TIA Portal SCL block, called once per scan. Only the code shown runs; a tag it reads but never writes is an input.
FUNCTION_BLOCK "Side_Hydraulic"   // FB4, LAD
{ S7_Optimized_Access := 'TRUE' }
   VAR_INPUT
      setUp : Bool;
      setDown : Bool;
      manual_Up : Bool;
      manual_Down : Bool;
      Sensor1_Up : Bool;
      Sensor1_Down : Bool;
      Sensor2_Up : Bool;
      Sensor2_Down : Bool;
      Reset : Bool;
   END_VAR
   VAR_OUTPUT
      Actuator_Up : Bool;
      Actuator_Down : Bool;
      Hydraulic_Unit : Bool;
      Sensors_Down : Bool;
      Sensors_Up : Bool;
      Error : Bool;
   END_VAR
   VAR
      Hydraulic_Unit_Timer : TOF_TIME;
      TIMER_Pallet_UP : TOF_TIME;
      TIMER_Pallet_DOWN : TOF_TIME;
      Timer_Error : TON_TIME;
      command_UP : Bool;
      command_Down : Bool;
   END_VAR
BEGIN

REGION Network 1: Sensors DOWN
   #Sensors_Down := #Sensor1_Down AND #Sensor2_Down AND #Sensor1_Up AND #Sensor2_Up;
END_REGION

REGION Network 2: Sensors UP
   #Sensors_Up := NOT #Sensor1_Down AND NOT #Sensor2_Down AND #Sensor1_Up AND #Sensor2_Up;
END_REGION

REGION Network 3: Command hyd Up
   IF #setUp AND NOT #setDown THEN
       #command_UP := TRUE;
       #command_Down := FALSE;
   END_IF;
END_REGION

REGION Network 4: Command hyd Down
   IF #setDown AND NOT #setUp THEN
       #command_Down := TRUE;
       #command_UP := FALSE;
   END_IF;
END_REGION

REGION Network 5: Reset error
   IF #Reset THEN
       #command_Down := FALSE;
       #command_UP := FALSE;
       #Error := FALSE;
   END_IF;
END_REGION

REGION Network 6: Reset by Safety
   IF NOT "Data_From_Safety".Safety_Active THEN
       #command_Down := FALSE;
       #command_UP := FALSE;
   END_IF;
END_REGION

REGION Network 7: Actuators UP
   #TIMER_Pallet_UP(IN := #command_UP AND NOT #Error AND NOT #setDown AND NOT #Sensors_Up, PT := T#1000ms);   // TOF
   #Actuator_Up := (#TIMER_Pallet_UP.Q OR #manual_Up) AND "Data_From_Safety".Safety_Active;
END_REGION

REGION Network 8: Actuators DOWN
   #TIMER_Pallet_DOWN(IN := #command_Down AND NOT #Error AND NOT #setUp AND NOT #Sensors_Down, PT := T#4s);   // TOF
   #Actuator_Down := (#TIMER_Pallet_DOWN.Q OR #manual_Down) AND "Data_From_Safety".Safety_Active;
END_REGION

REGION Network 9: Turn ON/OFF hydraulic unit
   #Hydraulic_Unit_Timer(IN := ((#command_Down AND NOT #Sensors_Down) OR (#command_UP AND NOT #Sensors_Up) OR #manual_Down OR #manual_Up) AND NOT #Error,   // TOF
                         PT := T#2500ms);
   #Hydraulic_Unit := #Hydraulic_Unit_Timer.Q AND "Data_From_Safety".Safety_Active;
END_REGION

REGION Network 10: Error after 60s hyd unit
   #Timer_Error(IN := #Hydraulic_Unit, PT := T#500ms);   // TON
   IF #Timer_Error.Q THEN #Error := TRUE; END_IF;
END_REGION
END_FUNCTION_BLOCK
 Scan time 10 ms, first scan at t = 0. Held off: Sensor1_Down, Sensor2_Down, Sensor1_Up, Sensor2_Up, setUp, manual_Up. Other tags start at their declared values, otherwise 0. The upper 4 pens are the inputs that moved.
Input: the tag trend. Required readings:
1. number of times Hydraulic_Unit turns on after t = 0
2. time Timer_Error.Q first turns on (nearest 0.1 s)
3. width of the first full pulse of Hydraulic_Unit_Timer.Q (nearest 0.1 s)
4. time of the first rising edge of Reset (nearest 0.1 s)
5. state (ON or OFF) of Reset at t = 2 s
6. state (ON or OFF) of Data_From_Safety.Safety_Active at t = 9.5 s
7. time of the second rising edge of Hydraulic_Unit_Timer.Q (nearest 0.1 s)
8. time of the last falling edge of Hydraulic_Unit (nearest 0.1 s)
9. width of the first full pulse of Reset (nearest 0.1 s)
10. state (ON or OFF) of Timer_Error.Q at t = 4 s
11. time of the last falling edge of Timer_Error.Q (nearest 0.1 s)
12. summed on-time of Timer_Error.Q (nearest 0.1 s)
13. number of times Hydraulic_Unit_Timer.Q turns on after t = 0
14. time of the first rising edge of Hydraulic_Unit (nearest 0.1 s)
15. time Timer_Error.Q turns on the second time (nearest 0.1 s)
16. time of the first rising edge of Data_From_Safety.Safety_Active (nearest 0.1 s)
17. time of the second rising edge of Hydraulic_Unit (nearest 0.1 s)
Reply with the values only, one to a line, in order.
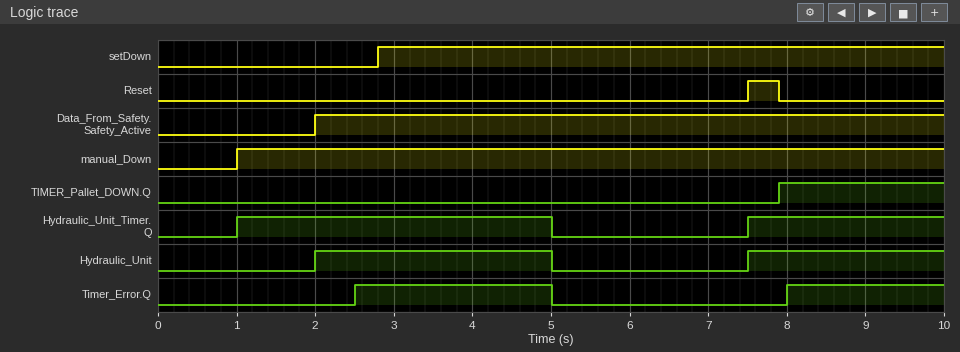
2
2.5 s
4.0 s
7.5 s
OFF
ON
7.5 s
5.0 s
0.4 s
ON
5.0 s
4.5 s
2
2.0 s
8.0 s
2.0 s
7.5 s
